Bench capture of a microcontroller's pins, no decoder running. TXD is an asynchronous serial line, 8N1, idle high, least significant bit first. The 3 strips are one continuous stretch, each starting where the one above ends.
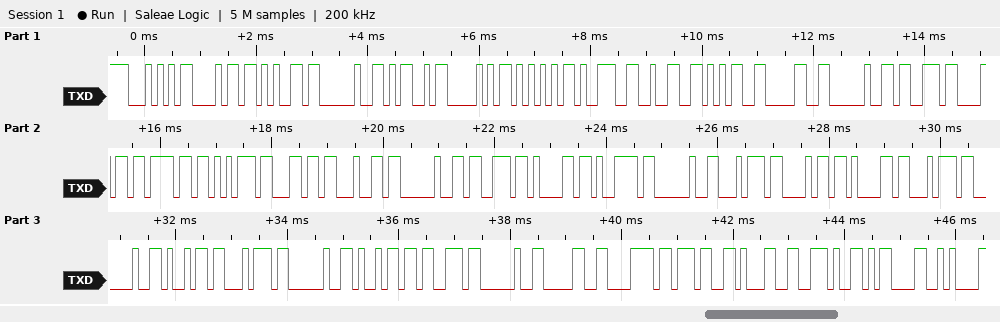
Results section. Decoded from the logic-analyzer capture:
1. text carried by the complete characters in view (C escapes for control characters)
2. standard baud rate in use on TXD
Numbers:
"The MPU9250 should say that it is 0x71.\r\n"
9600 baud
